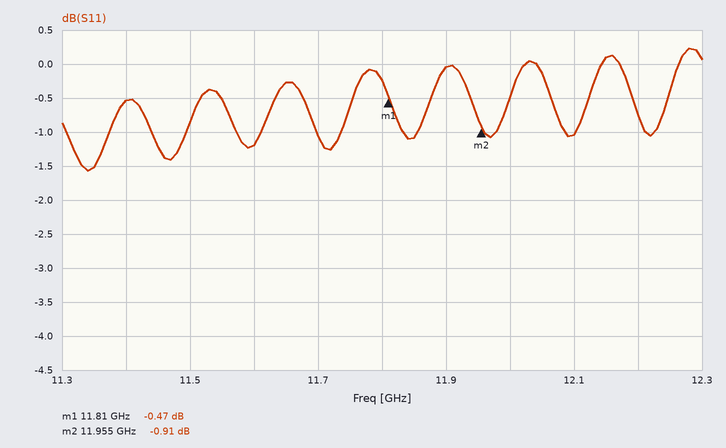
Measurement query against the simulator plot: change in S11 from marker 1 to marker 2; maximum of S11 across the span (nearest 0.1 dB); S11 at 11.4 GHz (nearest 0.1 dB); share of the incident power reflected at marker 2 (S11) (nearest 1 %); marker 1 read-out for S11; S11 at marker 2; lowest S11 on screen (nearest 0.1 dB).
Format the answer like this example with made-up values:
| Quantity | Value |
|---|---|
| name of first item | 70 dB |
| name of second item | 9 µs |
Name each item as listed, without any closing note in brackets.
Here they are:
| Quantity | Value |
|---|---|
| change in S11 from marker 1 to marker 2 | -0.44 dB |
| maximum of S11 across the span | 0.2 dB |
| S11 at 11.4 GHz | -0.5 dB |
| share of the incident power reflected at marker 2 (S11) | 81 % |
| marker 1 read-out for S11 | -0.47 dB |
| S11 at marker 2 | -0.91 dB |
| lowest S11 on screen | -1.6 dB |
